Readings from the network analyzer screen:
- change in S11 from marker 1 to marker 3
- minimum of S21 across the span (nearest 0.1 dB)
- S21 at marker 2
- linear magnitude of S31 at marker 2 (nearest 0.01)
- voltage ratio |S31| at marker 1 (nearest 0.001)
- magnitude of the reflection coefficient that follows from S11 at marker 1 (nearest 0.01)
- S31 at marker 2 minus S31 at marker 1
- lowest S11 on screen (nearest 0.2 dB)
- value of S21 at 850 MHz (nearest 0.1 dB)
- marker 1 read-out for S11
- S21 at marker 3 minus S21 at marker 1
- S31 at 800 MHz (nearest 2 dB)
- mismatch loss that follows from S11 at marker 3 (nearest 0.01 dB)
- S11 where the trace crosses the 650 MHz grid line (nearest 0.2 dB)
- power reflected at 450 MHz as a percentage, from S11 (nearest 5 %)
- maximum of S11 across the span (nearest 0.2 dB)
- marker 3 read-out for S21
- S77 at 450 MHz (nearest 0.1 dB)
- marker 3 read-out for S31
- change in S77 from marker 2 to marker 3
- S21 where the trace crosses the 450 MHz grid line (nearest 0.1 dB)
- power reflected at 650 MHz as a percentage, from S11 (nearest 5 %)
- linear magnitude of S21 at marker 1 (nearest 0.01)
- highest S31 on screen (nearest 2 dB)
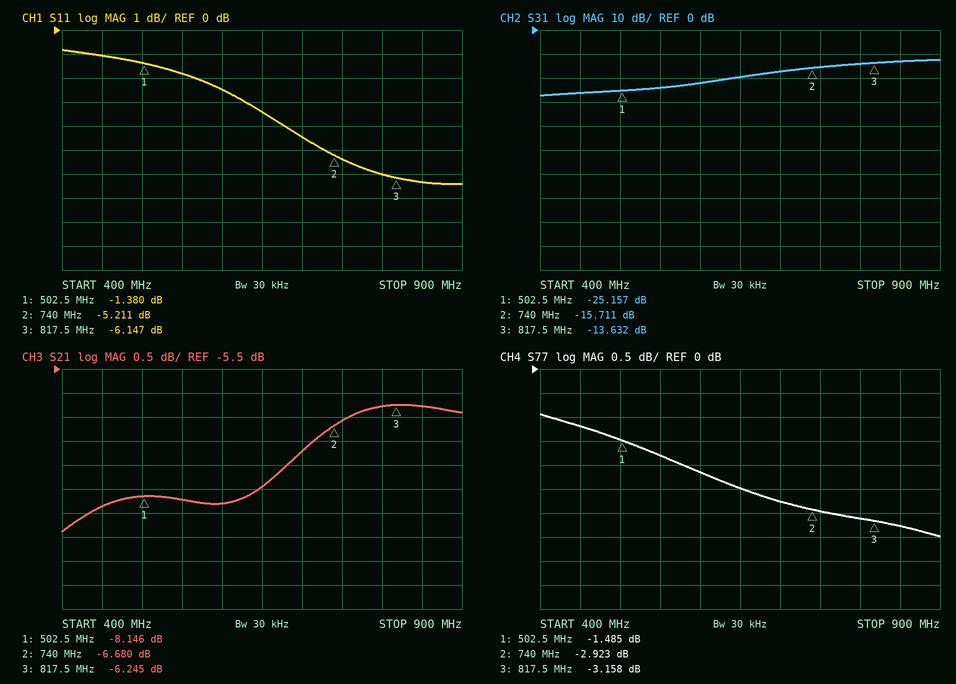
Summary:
-4.767 dB
-8.9 dB
-6.680 dB
0.16
0.055
0.85
9.446 dB
-6.4 dB
-6.3 dB
-1.380 dB
1.901 dB
-14 dB
1.21 dB
-3.4 dB
80 %
-0.8 dB
-6.245 dB
-1.2 dB
-13.632 dB
-0.235 dB
-8.4 dB
45 %
0.39
-12 dB
